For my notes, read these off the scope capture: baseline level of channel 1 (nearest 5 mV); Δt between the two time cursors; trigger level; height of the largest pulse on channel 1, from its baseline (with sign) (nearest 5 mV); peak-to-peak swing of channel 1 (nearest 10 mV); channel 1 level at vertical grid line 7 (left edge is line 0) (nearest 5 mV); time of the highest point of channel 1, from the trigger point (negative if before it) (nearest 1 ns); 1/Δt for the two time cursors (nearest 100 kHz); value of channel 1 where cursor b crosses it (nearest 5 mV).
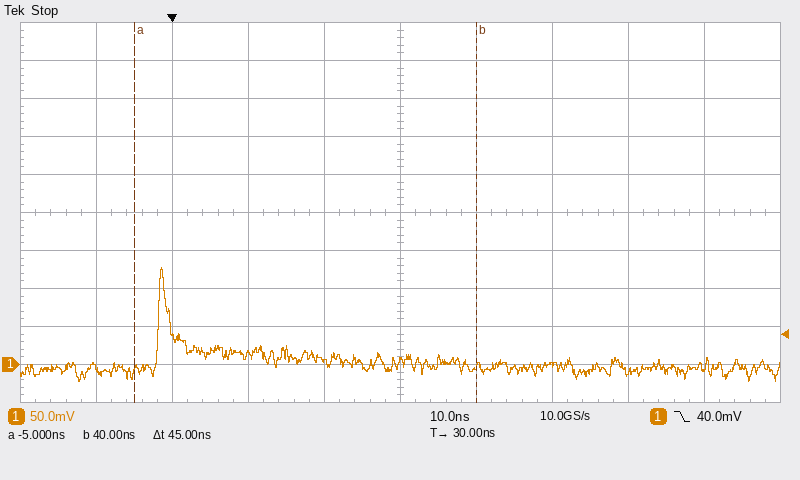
-5 mV
45 ns
40.0 mV
+130 mV
150 mV
0 mV
-1 ns
22.2 MHz
0 mV
